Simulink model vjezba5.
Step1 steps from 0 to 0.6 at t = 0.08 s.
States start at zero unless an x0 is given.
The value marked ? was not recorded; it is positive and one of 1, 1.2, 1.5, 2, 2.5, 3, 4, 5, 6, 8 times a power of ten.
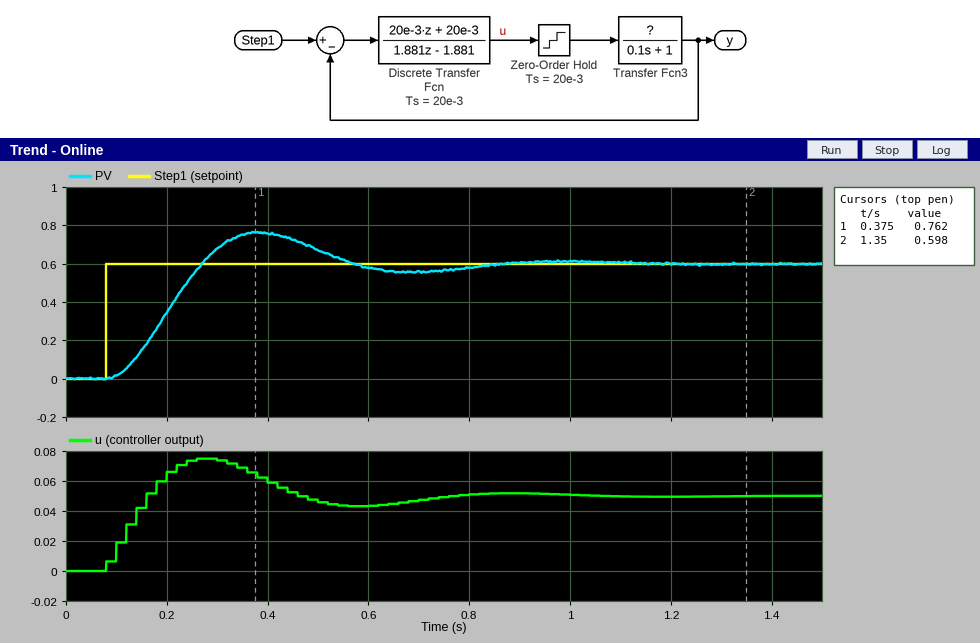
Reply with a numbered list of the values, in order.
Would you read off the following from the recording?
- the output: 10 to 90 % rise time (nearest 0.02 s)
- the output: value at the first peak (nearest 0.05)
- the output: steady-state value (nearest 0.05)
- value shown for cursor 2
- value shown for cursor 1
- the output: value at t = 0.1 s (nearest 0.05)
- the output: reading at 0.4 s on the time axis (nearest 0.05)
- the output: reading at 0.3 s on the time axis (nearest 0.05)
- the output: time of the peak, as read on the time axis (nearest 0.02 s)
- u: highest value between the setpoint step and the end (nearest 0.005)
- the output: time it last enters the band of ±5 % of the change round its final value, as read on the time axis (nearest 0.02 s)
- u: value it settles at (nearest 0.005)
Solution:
1. 0.12 s
2. 0.75
3. 0.60
4. 0.598
5. 0.762
6. 0.00
7. 0.75
8. 0.70
9. 0.38 s
10. 0.075
11. 0.76 s
12. 0.050
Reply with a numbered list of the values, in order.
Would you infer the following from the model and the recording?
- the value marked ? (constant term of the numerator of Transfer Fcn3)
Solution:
1. 12
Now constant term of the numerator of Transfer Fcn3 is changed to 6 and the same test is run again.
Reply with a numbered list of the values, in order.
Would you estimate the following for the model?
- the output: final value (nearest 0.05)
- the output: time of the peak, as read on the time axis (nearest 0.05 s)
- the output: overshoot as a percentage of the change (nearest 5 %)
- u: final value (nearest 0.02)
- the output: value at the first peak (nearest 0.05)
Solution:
1. 0.60
2. 0.55 s
3. 10 %
4. 0.10
5. 0.65
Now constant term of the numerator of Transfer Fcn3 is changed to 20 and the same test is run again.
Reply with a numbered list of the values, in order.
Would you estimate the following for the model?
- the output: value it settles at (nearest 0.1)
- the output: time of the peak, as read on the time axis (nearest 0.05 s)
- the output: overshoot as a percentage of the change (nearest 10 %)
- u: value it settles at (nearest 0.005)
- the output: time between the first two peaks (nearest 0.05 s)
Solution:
1. 0.6
2. 0.30 s
3. 40 %
4. 0.030
5. 0.45 s
